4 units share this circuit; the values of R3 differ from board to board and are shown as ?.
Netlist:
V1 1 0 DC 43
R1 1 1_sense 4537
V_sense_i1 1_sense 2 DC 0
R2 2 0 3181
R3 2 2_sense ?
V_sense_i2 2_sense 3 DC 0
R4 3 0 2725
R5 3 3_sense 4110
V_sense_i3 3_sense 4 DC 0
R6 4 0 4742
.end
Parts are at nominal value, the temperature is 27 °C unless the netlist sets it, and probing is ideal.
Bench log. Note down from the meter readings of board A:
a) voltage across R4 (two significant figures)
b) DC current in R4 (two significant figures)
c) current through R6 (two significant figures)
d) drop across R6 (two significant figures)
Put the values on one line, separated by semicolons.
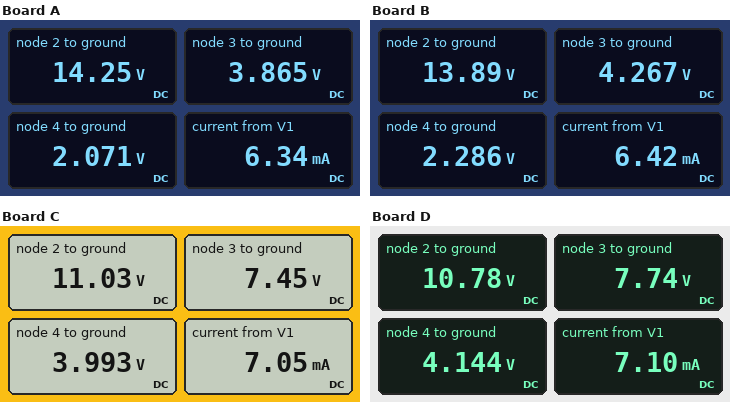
3.9 V; 1.4 mA; 440 µA; 2.1 V
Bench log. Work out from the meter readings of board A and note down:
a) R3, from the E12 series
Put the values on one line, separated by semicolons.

5.6 kΩ
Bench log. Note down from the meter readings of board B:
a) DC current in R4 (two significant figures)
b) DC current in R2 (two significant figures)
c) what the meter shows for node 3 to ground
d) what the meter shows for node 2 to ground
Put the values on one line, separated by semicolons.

1.6 mA; 4.4 mA; 4.267 V; 13.89 V
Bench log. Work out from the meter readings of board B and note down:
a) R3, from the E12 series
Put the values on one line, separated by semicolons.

4.7 kΩ
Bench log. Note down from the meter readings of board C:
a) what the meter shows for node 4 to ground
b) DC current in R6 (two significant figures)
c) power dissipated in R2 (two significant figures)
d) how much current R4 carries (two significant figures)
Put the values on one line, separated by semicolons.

3.993 V; 840 µA; 38 mW; 2.7 mA
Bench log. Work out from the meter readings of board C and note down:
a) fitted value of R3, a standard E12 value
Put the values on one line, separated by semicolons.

1 kΩ
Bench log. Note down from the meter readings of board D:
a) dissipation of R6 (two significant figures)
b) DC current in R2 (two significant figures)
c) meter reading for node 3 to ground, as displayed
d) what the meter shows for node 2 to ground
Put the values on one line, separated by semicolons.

3.6 mW; 3.4 mA; 7.74 V; 10.78 V
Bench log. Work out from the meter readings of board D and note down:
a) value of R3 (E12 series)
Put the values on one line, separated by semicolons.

820 Ω
